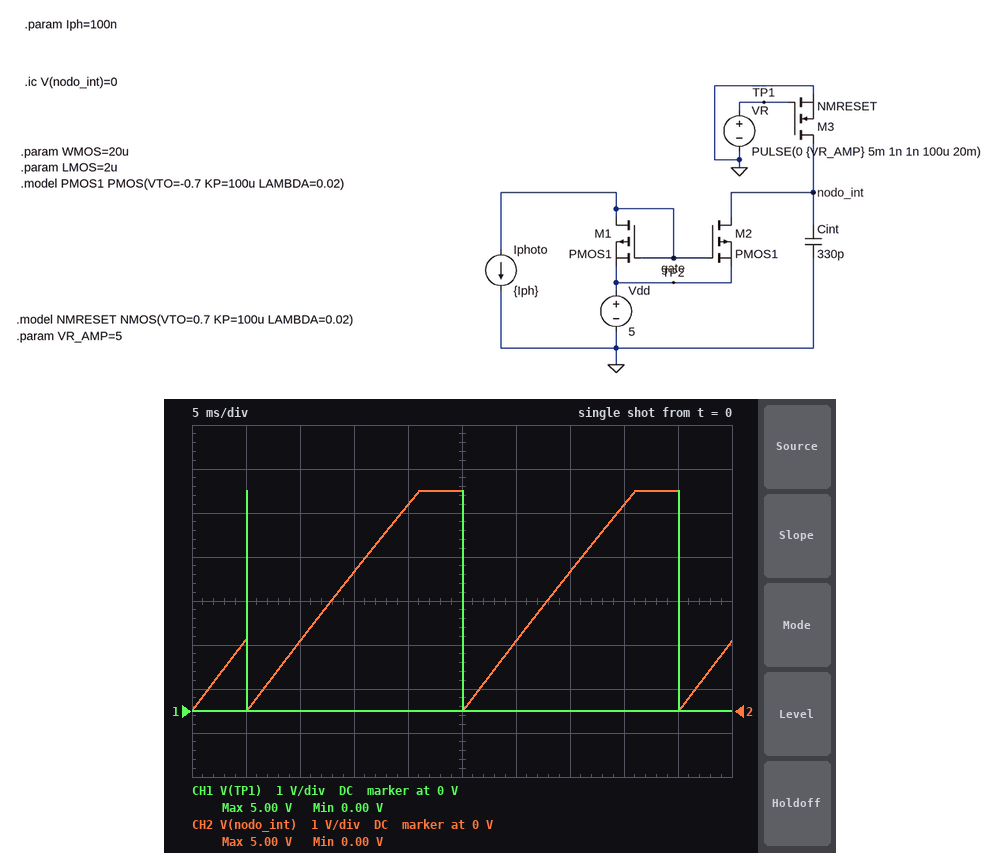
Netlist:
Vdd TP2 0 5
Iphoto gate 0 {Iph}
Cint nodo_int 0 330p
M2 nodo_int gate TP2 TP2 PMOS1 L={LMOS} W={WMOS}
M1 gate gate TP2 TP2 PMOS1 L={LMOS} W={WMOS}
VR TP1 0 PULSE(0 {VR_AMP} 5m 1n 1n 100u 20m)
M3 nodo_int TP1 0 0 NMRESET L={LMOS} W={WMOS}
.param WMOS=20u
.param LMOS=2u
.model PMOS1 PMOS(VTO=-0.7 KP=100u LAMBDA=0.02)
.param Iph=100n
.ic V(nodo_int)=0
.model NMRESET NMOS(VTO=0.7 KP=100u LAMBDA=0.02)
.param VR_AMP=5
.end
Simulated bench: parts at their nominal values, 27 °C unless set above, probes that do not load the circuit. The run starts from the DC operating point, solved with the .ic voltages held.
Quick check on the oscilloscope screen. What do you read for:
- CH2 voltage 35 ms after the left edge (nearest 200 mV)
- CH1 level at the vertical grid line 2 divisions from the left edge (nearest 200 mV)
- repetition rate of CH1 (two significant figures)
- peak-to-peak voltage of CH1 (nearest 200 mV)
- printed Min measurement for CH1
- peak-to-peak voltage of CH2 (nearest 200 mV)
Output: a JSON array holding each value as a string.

["3.2 V", "0 V", "50 Hz", "5.0 V", "0.00 V", "5.0 V"]
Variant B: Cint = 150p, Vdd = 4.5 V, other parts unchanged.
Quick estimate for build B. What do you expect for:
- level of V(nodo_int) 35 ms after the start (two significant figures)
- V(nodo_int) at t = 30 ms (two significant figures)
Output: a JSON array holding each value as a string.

["4.5 V", "3.4 V"]
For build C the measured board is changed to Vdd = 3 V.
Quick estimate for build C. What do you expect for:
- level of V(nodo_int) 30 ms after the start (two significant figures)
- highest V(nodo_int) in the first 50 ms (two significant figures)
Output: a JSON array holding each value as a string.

["1.5 V", "3.0 V"]
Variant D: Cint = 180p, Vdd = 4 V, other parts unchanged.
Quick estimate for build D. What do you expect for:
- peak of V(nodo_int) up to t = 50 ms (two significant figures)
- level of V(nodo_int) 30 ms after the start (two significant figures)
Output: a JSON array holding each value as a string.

["4.0 V", "2.8 V"]
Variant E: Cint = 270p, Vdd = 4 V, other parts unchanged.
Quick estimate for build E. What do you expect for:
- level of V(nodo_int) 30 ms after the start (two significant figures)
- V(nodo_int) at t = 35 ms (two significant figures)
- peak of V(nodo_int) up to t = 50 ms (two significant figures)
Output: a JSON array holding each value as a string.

["1.9 V", "3.8 V", "4.0 V"]
